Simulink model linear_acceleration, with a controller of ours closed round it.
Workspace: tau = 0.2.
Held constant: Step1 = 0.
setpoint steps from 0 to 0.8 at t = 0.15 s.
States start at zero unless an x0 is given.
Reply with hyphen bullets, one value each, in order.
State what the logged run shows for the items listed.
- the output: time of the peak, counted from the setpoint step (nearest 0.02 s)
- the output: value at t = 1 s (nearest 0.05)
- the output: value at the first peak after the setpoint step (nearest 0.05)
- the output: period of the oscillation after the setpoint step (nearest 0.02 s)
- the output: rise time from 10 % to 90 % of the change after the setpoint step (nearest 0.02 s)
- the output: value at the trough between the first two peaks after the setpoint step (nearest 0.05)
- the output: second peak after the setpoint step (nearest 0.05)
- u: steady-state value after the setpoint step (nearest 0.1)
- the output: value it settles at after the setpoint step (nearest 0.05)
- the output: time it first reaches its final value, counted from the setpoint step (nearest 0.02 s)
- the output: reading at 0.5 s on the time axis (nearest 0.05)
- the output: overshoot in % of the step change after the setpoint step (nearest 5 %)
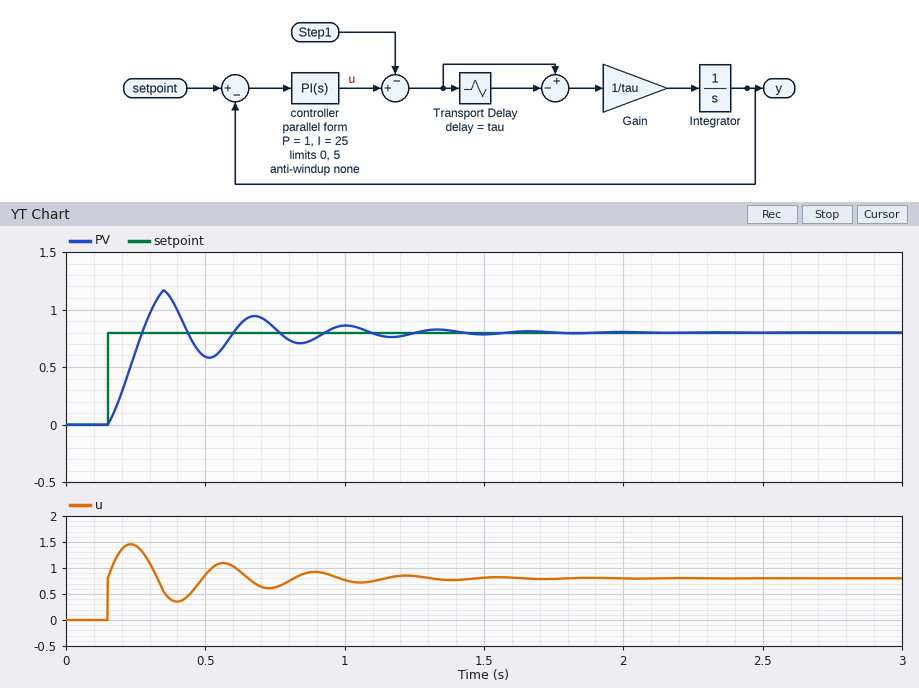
- 0.20 s
- 0.85
- 1.15
- 0.32 s
- 0.10 s
- 0.60
- 0.95
- 0.8
- 0.80
- 0.12 s
- 0.60
- 45 %
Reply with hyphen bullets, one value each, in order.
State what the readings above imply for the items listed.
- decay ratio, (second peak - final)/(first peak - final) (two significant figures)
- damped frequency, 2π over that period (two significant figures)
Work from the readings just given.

- 0.43
- 20 rad/s
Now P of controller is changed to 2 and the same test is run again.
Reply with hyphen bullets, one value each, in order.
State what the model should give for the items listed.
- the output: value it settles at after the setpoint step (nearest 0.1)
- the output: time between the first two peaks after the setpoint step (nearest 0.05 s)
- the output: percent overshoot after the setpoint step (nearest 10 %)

- 0.8
- 0.25 s
- 30 %
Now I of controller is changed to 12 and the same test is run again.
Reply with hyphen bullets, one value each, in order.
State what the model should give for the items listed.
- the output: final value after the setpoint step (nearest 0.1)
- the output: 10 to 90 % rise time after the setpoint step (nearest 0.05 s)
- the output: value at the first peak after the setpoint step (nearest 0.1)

- 0.8
- 0.15 s
- 0.9
